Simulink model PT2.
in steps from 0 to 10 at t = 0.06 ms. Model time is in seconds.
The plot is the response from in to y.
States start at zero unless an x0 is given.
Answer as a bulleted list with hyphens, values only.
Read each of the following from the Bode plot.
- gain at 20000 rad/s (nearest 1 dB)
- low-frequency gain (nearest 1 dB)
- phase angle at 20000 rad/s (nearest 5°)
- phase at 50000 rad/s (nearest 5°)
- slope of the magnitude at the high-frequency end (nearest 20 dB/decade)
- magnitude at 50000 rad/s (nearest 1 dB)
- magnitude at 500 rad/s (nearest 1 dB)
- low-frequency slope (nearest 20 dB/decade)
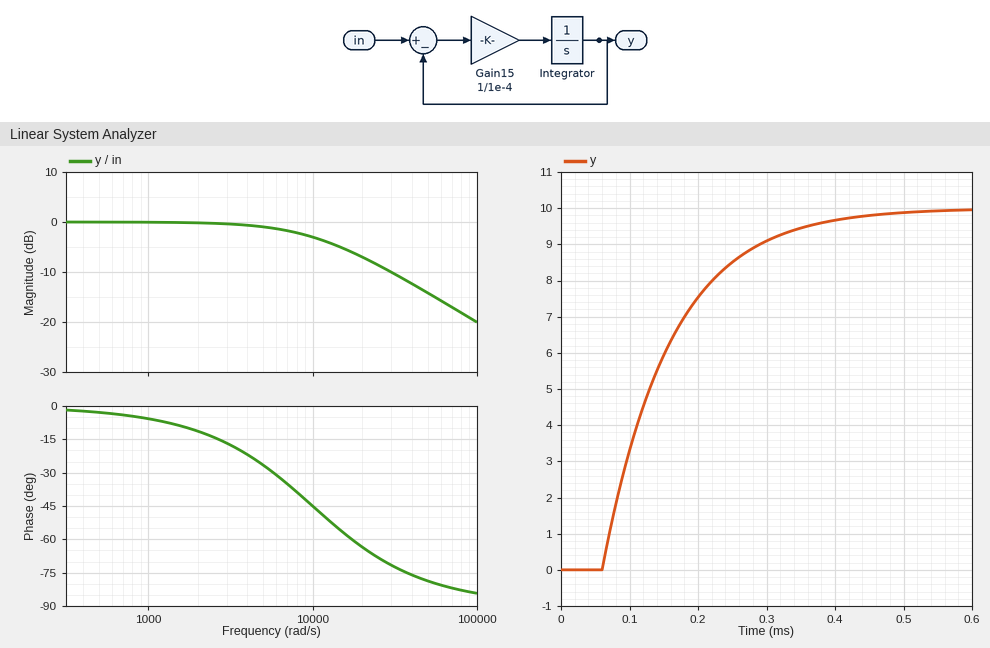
- -7 dB
- 0 dB
- -65°
- -80°
- -20 dB/decade
- -14 dB
- 0 dB
- 0 dB/decade
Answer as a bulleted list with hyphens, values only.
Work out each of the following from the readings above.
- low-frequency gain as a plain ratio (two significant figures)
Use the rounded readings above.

- 1.0
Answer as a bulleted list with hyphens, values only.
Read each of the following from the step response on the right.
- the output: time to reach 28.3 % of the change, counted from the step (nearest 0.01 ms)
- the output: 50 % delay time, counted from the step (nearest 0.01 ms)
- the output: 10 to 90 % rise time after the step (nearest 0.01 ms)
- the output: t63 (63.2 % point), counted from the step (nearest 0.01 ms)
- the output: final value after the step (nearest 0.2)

- 0.03 ms
- 0.07 ms
- 0.22 ms
- 0.10 ms
- 10.0
